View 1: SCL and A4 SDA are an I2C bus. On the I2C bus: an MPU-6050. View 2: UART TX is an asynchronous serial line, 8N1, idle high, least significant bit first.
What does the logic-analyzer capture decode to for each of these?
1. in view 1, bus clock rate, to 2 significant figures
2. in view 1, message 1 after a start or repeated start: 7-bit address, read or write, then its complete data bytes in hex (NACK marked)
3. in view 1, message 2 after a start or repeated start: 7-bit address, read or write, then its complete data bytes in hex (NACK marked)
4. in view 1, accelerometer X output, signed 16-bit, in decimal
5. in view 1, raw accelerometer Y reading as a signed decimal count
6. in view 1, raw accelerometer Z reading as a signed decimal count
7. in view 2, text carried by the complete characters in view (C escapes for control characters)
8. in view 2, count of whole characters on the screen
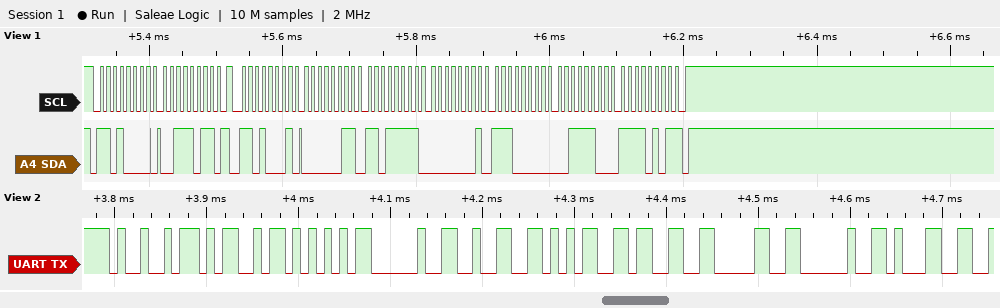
100 kHz
0x68 write: 3B
0x68 read: 03 DF 01 E0 3C F5 NACK
991
480
15605
"IMU 2530 1"
10
